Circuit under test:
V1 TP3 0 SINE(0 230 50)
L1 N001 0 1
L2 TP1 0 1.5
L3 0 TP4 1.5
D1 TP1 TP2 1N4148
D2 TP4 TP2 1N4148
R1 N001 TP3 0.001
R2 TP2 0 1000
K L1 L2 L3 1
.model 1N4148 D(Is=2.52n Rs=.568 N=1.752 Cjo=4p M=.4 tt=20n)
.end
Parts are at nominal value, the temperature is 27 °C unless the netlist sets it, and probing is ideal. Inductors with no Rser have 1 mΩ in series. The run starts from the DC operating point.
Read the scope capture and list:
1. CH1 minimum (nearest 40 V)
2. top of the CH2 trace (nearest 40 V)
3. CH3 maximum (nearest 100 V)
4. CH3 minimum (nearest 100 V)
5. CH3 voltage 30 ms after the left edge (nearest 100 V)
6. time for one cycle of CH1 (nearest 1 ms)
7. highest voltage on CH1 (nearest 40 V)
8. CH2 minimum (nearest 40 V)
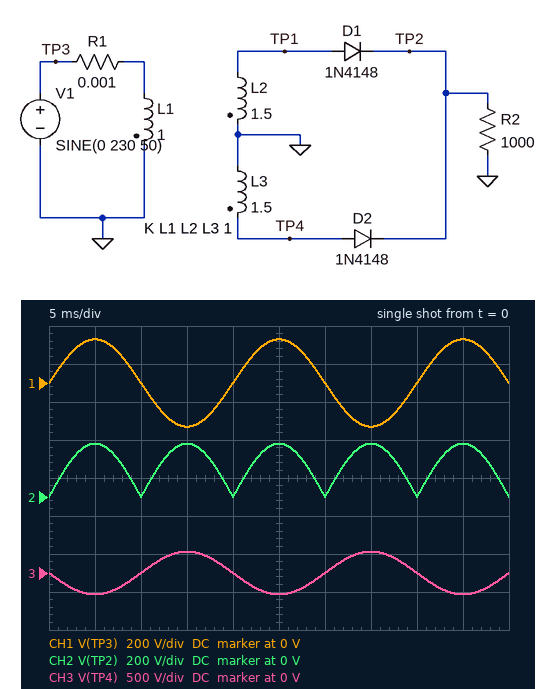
-240 V
280 V
300 V
-300 V
0 V
20 ms
240 V
0 V
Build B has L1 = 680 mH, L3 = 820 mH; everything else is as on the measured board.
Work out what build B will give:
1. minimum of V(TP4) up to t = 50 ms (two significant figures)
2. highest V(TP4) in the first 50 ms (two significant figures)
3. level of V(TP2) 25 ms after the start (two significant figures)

-250 V
250 V
340 V
